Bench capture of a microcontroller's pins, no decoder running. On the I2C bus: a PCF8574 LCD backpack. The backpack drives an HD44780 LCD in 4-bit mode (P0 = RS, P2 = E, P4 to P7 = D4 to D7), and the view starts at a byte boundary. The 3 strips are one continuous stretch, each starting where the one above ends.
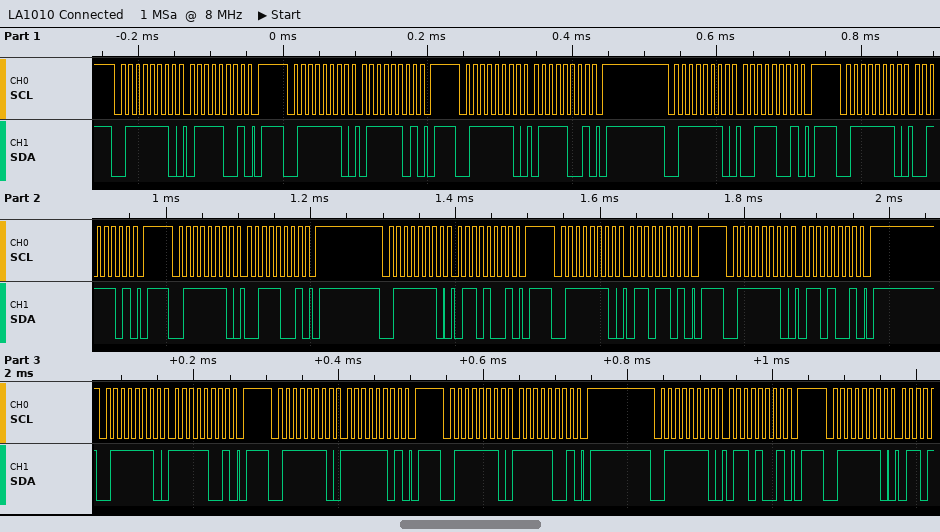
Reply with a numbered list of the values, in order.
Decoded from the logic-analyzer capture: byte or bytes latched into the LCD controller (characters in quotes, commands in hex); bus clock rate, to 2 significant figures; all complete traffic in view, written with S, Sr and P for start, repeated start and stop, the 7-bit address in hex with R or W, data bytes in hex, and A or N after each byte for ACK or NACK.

1. 's' 'o'
2. 100 kHz
3. S 3FW A 79 A P S 3FW A 7D A P S 3FW A 79 A P S 3FW A 39 A P S 3FW A 3D A P S 3FW A 39 A P S 3FW A 69 A P S 3FW A 6D A P S 3FW A 69 A P S 3FW A F9 A P S 3FW A FD A P S 3FW A F9 A P S 3FW A 69 A P S 3FW A
